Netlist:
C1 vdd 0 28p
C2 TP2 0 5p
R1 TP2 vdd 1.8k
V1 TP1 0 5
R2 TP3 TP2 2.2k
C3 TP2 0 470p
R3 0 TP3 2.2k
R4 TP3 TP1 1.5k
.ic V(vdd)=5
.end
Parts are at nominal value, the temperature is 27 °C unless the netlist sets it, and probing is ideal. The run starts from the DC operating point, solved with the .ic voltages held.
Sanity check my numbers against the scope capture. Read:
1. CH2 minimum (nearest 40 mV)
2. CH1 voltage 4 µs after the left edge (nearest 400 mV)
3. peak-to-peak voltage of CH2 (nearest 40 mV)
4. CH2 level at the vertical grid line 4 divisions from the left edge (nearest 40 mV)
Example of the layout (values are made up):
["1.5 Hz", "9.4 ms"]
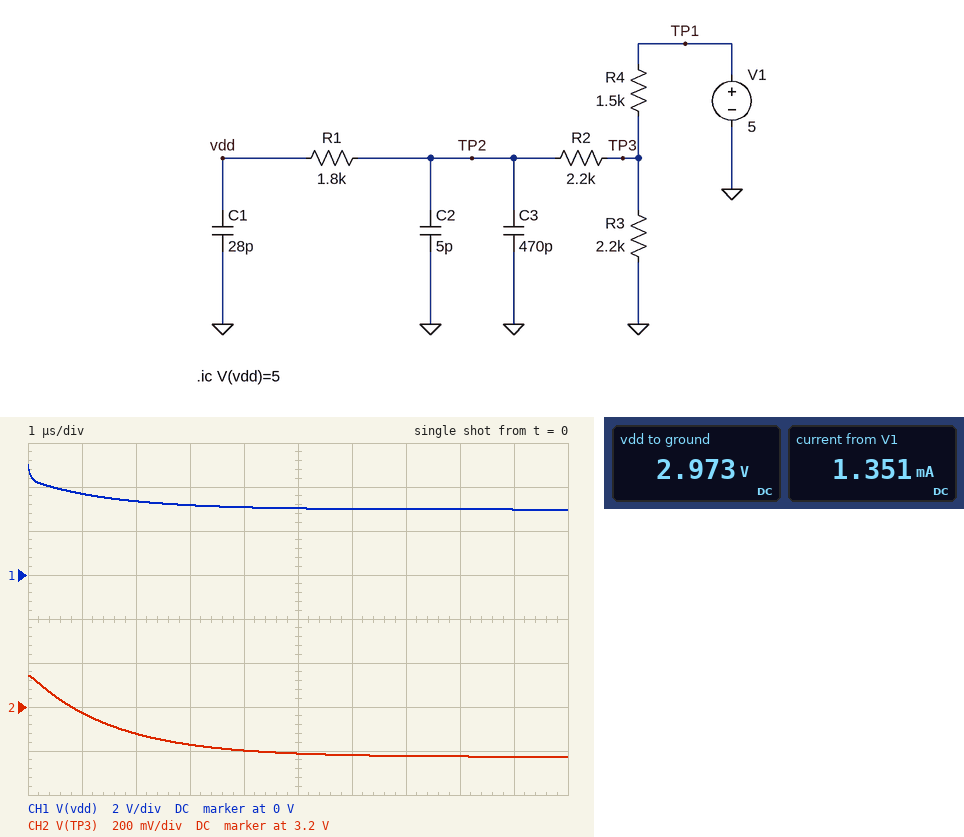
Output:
["2.96 V", "3.2 V", "360 mV", "3.00 V"]
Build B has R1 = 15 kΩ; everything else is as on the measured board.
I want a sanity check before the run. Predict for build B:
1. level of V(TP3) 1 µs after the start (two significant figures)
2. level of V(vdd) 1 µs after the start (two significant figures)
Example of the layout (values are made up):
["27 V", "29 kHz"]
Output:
["3.0 V", "3.4 V"]
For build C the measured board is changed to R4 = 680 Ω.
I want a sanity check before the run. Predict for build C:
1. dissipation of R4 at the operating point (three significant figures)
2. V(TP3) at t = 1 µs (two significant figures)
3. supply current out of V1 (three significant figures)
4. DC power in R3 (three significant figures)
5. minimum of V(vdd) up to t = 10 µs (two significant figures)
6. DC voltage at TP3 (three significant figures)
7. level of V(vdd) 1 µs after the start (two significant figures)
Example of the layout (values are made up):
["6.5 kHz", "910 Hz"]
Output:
["2.05 mW", "3.9 V", "1.74 mA", "6.63 mW", "3.8 V", "3.82 V", "4.2 V"]
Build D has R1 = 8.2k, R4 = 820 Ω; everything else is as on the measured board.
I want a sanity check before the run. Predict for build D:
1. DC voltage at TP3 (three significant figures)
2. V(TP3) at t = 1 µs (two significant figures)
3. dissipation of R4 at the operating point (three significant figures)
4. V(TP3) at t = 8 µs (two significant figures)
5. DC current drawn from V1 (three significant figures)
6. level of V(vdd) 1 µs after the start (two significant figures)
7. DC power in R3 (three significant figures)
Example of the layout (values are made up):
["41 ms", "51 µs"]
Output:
["3.64 V", "3.7 V", "2.25 mW", "3.6 V", "1.66 mA", "3.9 V", "6.03 mW"]
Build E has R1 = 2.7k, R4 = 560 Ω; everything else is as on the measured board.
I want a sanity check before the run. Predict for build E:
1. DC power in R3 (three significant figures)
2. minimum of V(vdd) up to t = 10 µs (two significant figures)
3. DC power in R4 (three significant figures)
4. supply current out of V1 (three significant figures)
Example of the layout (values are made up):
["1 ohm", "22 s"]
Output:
["7.22 mW", "4.0 V", "1.84 mW", "1.81 mA"]
